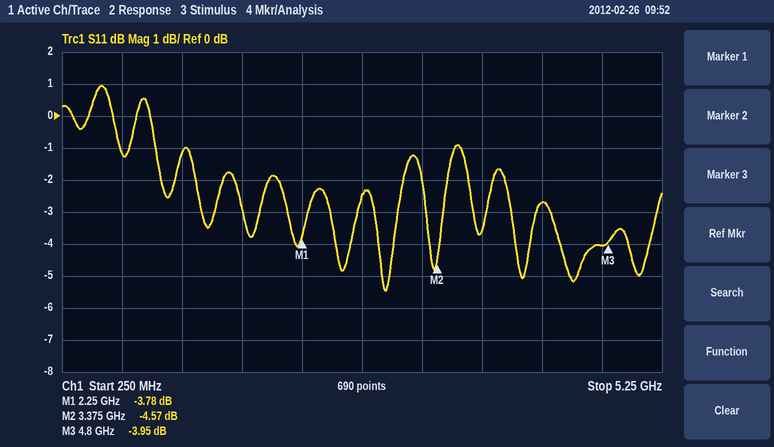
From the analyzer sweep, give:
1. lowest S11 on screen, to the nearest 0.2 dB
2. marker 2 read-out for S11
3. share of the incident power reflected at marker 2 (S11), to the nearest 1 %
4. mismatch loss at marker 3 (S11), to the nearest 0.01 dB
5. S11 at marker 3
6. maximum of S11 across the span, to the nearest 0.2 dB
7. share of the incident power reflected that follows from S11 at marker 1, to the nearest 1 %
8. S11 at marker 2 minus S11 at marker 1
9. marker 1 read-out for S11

-5.4 dB
-4.57 dB
35 %
2.24 dB
-3.95 dB
1.0 dB
42 %
-0.79 dB
-3.78 dB
